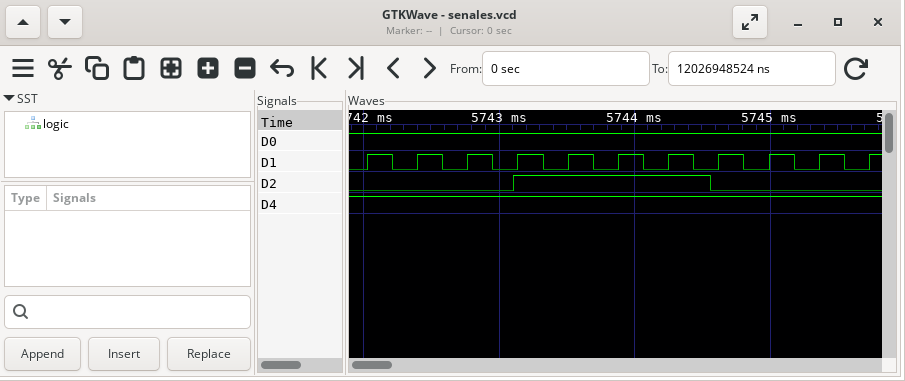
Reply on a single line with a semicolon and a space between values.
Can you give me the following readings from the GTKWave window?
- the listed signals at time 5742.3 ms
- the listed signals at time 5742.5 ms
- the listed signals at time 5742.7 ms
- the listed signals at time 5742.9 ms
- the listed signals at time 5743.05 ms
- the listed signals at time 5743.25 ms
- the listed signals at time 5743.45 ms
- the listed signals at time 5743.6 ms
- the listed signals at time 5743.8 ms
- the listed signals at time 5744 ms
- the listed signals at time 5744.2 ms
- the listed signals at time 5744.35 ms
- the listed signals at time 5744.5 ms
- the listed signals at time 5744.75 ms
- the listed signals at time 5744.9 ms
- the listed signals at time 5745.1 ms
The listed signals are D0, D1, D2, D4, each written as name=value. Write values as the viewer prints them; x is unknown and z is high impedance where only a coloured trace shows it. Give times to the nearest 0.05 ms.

D0=1, D1=0, D2=0, D4=1; D0=1, D1=1, D2=0, D4=1; D0=1, D1=0, D2=0, D4=1; D0=1, D1=1, D2=0, D4=1; D0=1, D1=0, D2=0, D4=1; D0=1, D1=1, D2=1, D4=1; D0=1, D1=0, D2=1, D4=1; D0=1, D1=1, D2=1, D4=1; D0=1, D1=0, D2=1, D4=1; D0=1, D1=1, D2=1, D4=1; D0=1, D1=0, D2=1, D4=1; D0=1, D1=1, D2=1, D4=1; D0=1, D1=0, D2=1, D4=1; D0=1, D1=1, D2=0, D4=1; D0=1, D1=0, D2=0, D4=1; D0=1, D1=1, D2=0, D4=1
